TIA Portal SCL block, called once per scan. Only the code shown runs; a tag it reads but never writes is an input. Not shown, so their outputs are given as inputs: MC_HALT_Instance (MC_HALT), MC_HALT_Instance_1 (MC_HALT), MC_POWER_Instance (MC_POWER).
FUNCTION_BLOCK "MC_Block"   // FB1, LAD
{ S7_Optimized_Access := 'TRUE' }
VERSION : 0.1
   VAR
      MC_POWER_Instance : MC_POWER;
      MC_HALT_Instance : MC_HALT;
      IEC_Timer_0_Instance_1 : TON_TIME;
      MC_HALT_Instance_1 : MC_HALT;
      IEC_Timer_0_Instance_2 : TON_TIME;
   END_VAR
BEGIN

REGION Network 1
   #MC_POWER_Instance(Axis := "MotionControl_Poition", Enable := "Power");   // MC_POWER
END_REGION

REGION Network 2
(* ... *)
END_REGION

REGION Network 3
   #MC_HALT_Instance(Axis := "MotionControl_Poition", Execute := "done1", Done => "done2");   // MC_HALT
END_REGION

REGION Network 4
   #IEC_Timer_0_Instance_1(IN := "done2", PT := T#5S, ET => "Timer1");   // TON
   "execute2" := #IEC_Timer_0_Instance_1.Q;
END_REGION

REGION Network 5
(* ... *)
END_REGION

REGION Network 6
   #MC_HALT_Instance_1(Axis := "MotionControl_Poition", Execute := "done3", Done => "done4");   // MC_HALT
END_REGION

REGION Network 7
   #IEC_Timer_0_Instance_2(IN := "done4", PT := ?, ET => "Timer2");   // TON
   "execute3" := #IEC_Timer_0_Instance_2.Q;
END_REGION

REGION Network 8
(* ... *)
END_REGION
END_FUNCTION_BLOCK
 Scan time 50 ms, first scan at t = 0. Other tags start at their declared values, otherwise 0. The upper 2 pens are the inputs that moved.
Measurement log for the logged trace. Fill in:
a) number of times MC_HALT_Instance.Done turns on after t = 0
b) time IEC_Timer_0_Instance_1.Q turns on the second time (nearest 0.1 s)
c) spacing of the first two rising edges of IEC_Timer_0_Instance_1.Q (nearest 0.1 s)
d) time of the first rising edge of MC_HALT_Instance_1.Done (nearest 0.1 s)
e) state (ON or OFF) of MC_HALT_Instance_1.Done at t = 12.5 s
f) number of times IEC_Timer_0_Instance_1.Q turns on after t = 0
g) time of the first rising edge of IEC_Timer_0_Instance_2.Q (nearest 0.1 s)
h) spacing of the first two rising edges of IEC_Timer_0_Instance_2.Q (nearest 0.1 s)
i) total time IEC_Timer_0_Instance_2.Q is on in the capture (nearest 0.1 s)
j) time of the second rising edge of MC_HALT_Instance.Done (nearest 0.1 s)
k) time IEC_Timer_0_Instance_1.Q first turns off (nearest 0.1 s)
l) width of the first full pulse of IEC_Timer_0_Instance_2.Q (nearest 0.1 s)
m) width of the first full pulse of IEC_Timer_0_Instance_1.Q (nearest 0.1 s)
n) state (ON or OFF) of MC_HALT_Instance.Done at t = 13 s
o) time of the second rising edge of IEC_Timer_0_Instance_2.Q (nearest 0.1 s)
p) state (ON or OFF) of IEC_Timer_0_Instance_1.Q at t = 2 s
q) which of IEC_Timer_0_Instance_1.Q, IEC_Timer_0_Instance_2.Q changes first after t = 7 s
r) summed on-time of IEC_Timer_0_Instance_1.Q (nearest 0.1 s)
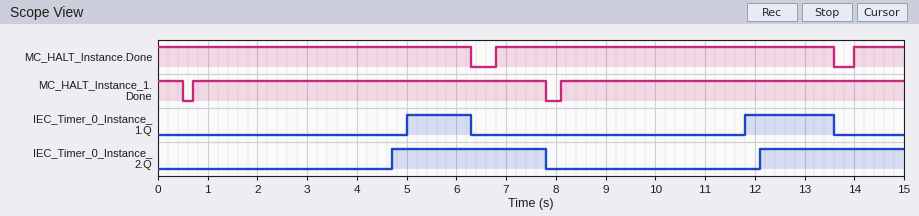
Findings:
2
11.8 s
6.8 s
0.7 s
ON
2
4.7 s
7.4 s
6.0 s
14.0 s
6.3 s
3.1 s
1.3 s
ON
12.1 s
OFF
IEC_Timer_0_Instance_2.Q
3.1 s
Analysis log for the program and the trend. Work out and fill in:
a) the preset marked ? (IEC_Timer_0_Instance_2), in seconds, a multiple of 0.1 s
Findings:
4.0 s
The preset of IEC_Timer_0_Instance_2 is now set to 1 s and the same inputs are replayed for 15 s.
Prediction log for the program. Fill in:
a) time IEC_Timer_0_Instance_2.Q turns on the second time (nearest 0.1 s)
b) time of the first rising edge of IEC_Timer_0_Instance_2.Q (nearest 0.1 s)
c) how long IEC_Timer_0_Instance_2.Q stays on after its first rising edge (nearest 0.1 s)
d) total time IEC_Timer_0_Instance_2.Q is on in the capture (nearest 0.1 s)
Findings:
9.1 s
1.7 s
6.1 s
12.0 s
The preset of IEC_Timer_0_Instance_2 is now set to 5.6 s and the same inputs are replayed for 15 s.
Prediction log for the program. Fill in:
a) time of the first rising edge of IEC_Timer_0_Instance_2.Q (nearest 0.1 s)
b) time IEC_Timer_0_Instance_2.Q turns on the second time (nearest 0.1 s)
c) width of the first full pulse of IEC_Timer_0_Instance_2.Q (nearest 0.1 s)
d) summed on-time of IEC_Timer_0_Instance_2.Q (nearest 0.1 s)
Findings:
6.3 s
13.7 s
1.5 s
2.8 s
